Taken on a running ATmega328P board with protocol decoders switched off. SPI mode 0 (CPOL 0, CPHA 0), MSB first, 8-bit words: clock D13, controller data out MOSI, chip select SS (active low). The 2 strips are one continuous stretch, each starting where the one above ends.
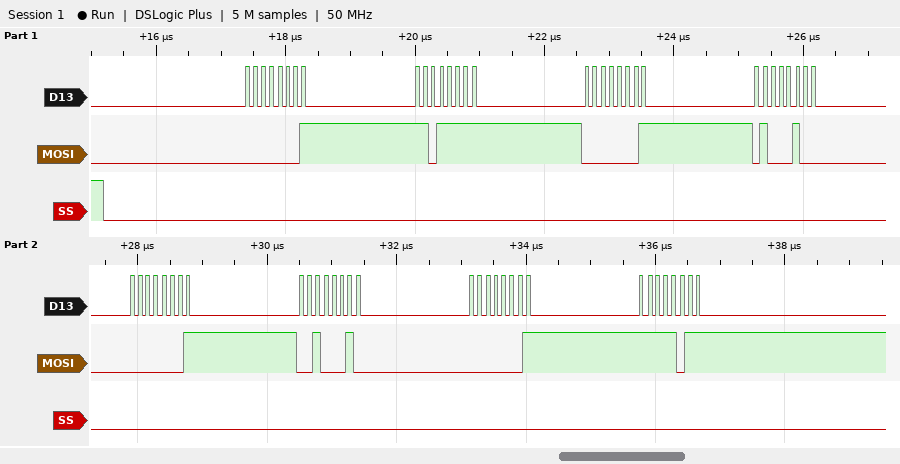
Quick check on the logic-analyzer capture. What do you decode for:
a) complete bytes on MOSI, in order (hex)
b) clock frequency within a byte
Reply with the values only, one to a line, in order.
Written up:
01 DF 01 44 01 22 01 FB
8 MHz
